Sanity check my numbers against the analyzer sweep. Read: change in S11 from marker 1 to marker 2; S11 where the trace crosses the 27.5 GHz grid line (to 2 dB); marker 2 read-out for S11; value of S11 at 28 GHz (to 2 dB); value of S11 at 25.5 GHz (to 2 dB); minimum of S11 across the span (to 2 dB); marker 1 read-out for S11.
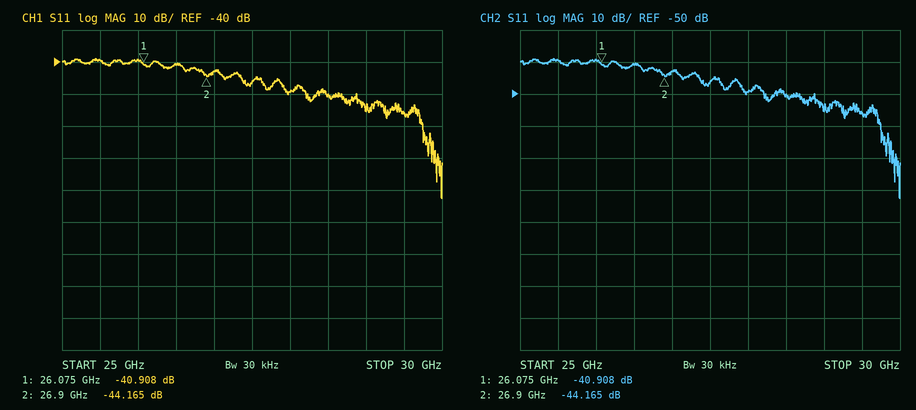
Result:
-3.257 dB
-46 dB
-44.165 dB
-50 dB
-40 dB
-82 dB
-40.908 dB
